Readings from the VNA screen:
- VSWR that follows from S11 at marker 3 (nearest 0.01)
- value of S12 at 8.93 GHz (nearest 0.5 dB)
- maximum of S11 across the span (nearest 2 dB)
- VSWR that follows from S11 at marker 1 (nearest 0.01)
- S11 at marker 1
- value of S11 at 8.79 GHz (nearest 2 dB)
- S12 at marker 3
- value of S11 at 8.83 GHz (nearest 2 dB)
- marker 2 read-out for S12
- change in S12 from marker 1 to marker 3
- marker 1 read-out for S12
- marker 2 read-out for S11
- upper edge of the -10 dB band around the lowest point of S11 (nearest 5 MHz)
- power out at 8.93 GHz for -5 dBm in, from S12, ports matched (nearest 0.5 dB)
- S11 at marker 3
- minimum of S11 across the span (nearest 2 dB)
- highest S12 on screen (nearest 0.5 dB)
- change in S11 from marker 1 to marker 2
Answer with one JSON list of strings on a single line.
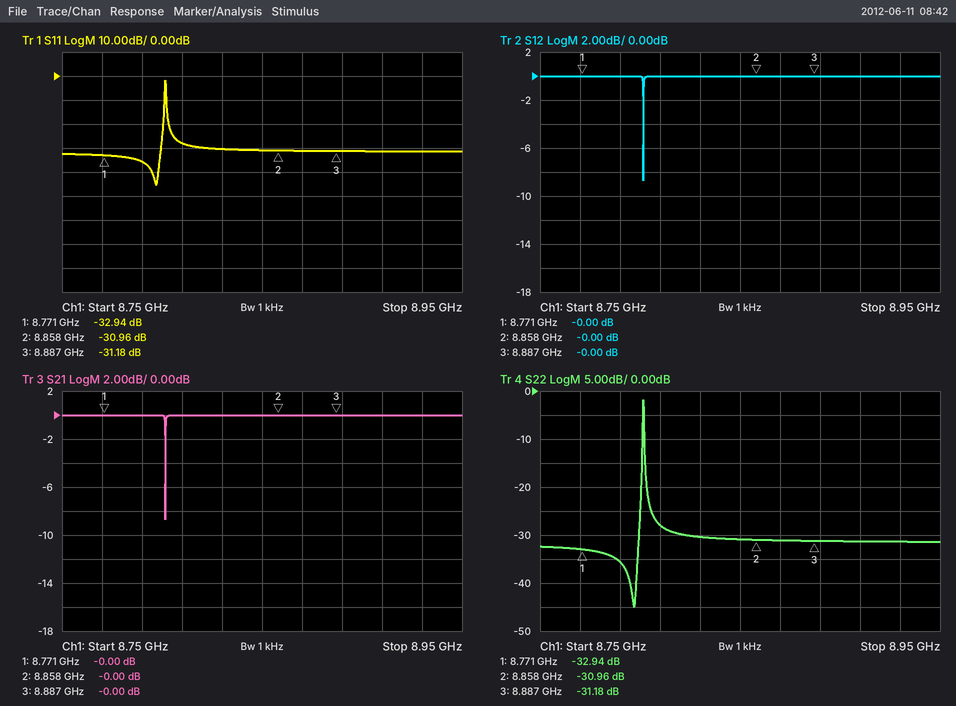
["1.06", "0.0 dB", "-2 dB", "1.05", "-32.94 dB", "-36 dB", "-0.00 dB", "-30 dB", "-0.00 dB", "0.00 dB", "-0.00 dB", "-30.96 dB", "8.800 GHz", "-5.0 dBm", "-31.18 dB", "-46 dB", "0.0 dB", "1.98 dB"]
